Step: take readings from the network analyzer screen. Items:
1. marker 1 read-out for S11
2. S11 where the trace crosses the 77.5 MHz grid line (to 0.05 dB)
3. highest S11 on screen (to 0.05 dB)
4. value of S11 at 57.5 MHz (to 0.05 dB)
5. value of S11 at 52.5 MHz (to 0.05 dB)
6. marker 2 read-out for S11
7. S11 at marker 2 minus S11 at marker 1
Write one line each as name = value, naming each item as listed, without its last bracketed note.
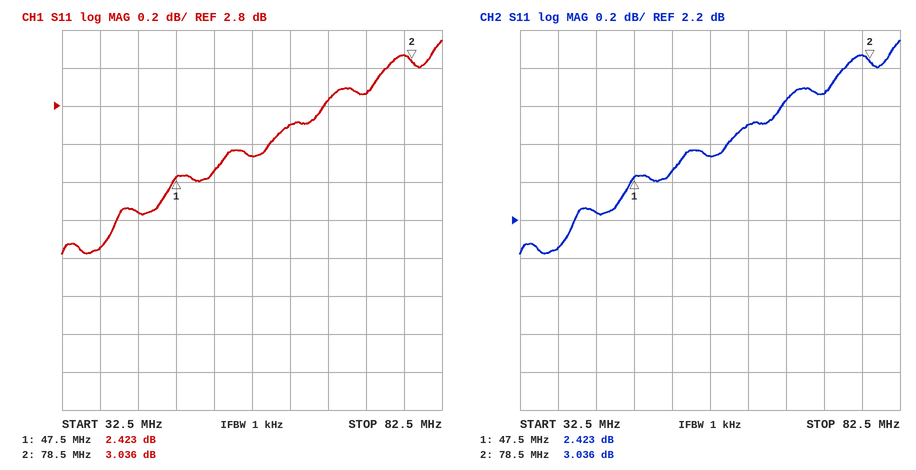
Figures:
marker 1 read-out for S11 = 2.423 dB
S11 where the trace crosses the 77.5 MHz grid line = 3.05 dB
highest S11 on screen = 3.15 dB
value of S11 at 57.5 MHz = 2.55 dB
value of S11 at 52.5 MHz = 2.45 dB
marker 2 read-out for S11 = 3.036 dB
S11 at marker 2 minus S11 at marker 1 = 0.613 dB
